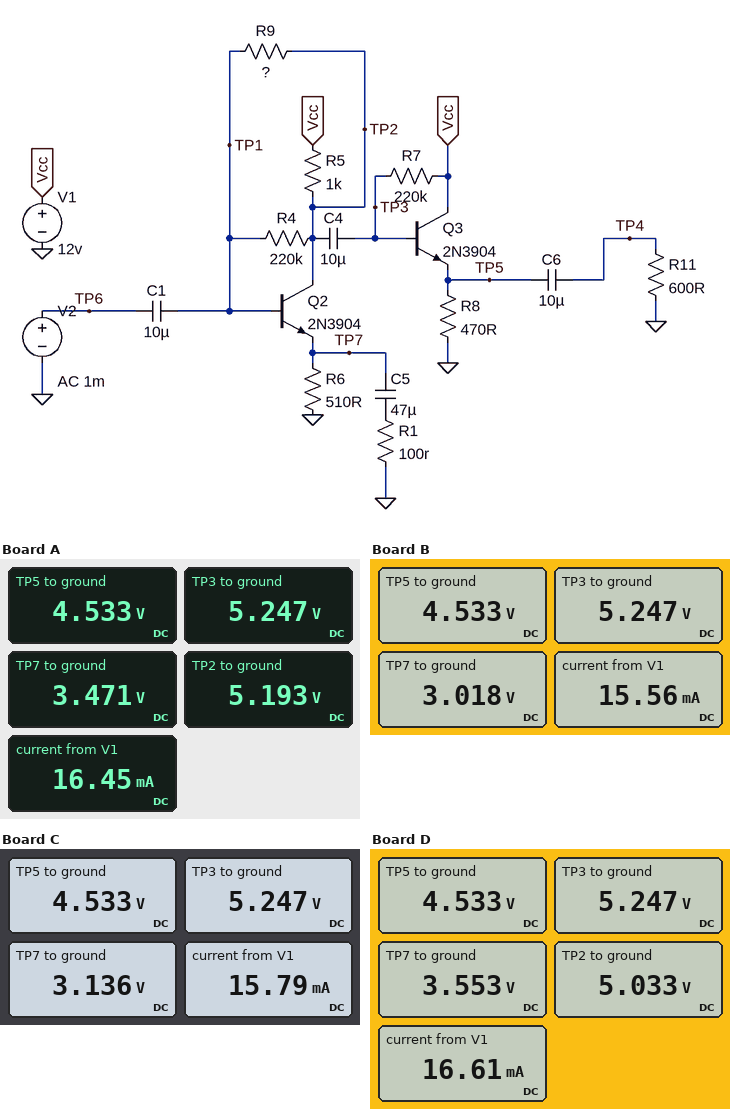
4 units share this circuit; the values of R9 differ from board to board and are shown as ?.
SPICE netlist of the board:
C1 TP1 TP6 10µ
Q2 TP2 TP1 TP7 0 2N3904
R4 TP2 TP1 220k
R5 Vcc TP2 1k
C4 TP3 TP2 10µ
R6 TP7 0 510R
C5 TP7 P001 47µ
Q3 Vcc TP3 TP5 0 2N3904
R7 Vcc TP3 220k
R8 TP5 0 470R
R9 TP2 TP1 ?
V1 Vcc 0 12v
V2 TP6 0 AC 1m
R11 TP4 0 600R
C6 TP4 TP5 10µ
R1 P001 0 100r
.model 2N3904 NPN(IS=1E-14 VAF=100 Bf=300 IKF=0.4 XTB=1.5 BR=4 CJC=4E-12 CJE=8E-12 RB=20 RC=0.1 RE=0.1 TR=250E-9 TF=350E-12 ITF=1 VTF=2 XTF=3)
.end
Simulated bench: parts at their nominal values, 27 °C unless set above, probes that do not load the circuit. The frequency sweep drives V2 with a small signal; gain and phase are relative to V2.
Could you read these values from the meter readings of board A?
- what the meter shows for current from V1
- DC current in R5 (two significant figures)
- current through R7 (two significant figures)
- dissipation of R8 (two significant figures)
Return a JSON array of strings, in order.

["16.45 mA", "6.8 mA", "31 µA", "44 mW"]
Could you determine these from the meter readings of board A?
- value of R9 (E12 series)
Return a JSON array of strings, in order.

["56 kΩ"]
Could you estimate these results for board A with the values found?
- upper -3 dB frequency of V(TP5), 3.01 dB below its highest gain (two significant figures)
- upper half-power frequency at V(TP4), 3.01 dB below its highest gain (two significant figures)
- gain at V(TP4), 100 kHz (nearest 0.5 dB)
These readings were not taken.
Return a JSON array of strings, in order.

["23 MHz", "23 MHz", "20.5 dB"]
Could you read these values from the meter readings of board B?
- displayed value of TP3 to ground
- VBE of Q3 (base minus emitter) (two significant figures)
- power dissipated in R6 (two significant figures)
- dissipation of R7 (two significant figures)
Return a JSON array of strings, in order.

["5.247 V", "710 mV", "18 mW", "210 µW"]
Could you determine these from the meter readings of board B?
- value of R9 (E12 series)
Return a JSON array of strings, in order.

["270 kΩ"]
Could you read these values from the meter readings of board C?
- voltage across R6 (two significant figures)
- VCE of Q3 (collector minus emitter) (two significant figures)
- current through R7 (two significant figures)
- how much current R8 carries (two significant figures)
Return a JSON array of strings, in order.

["3.1 V", "7.5 V", "31 µA", "9.6 mA"]
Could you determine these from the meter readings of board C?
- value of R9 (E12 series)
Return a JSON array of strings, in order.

["180 kΩ"]
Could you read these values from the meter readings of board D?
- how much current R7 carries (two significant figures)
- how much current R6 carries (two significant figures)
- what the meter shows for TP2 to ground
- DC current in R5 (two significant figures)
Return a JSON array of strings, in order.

["31 µA", "7.0 mA", "5.033 V", "7.0 mA"]
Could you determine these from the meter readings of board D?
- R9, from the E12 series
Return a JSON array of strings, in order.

["39 kΩ"]
